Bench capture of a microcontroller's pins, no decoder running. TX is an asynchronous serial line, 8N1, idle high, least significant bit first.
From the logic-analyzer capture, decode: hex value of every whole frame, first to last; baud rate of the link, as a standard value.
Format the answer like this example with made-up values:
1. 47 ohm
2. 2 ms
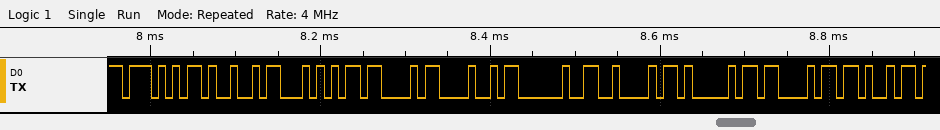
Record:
1. 0x57 0x49 0x54 0x43 0x48 0x20 0x42 0x41 0x43 0x4B
2. 115200 baud
